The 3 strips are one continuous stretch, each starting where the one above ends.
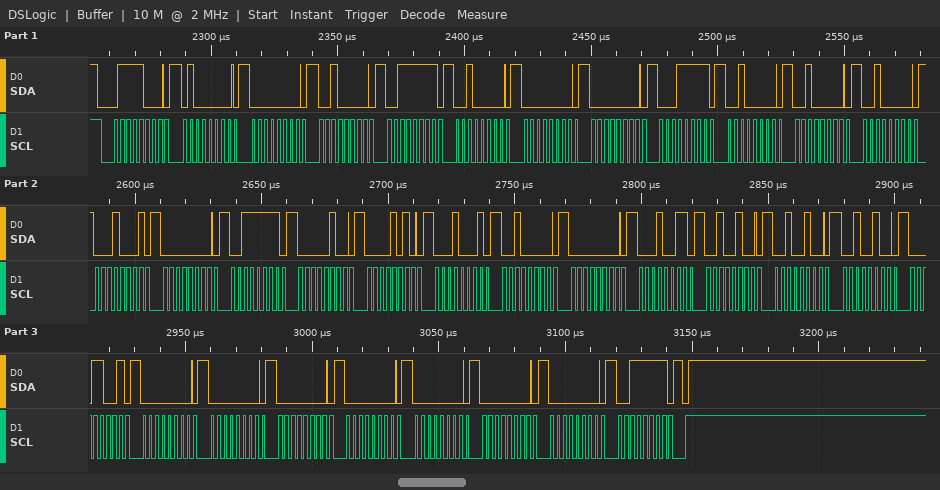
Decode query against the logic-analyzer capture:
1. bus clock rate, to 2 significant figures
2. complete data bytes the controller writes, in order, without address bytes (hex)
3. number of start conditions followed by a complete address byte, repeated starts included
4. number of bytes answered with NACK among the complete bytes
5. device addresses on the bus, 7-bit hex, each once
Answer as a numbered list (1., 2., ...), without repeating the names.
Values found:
1. 400 kHz
2. 40 00 20 3F 20 00 00 1F 20 20 20 11 00 3F 04 0A 11 20 00 13 24 24 24 19 00 00 00 00 00 00 00 3F
3. 1
4. 0
5. 0x3C
